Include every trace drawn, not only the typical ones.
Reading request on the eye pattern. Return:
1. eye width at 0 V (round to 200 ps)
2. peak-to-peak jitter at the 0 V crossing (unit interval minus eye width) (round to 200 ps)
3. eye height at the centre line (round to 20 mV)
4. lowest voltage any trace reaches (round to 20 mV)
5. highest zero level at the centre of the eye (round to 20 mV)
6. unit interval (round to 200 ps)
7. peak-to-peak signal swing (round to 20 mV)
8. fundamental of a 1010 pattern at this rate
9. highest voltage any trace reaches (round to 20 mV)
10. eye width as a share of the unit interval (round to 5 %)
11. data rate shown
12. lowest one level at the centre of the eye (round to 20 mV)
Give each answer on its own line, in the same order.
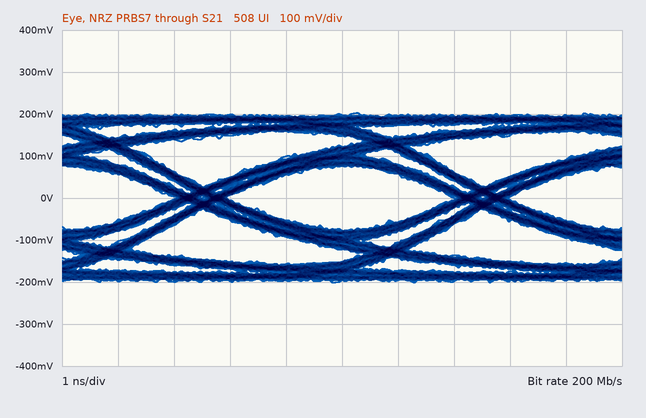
4.0 ns
1.0 ns
160 mV
-200 mV
-80 mV
5.0 ns
400 mV
100 MHz
200 mV
80 %
200 Mb/s
80 mV
